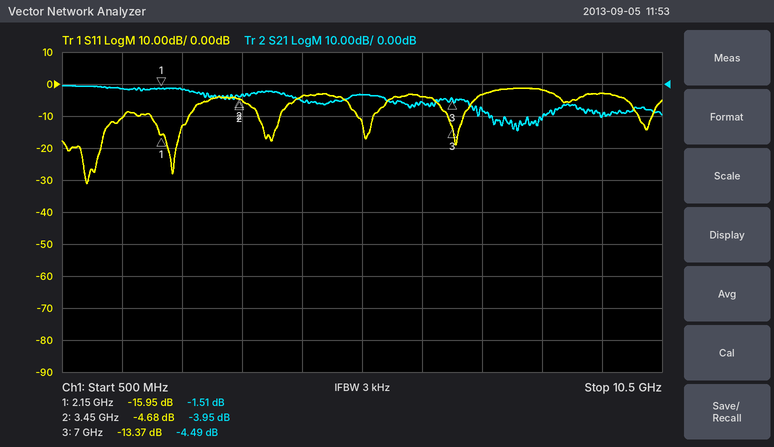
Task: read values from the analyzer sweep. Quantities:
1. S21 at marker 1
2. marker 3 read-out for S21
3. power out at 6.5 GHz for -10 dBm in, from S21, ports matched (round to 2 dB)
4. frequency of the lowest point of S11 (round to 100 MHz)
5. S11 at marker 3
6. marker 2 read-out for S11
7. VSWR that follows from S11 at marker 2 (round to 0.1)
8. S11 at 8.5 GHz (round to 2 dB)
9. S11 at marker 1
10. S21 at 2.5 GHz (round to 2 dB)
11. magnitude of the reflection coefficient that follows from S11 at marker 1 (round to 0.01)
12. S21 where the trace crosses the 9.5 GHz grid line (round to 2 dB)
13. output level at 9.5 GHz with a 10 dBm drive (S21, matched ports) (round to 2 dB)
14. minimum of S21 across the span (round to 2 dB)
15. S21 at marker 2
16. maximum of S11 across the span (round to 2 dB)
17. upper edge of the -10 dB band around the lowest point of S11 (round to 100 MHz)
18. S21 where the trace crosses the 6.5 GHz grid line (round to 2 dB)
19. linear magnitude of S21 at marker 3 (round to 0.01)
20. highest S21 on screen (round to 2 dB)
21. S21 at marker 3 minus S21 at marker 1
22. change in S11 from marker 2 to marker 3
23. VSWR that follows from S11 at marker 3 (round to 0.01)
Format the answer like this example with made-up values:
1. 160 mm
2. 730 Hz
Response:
1. -1.51 dB
2. -4.49 dB
3. -16 dBm
4. 900 MHz
5. -13.37 dB
6. -4.68 dB
7. 3.8
8. -2 dB
9. -15.95 dB
10. -2 dB
11. 0.16
12. -10 dB
13. 0 dBm
14. -14 dB
15. -3.95 dB
16. -2 dB
17. 1.5 GHz
18. -6 dB
19. 0.60
20. 0 dB
21. -2.98 dB
22. -8.69 dB
23. 1.55
